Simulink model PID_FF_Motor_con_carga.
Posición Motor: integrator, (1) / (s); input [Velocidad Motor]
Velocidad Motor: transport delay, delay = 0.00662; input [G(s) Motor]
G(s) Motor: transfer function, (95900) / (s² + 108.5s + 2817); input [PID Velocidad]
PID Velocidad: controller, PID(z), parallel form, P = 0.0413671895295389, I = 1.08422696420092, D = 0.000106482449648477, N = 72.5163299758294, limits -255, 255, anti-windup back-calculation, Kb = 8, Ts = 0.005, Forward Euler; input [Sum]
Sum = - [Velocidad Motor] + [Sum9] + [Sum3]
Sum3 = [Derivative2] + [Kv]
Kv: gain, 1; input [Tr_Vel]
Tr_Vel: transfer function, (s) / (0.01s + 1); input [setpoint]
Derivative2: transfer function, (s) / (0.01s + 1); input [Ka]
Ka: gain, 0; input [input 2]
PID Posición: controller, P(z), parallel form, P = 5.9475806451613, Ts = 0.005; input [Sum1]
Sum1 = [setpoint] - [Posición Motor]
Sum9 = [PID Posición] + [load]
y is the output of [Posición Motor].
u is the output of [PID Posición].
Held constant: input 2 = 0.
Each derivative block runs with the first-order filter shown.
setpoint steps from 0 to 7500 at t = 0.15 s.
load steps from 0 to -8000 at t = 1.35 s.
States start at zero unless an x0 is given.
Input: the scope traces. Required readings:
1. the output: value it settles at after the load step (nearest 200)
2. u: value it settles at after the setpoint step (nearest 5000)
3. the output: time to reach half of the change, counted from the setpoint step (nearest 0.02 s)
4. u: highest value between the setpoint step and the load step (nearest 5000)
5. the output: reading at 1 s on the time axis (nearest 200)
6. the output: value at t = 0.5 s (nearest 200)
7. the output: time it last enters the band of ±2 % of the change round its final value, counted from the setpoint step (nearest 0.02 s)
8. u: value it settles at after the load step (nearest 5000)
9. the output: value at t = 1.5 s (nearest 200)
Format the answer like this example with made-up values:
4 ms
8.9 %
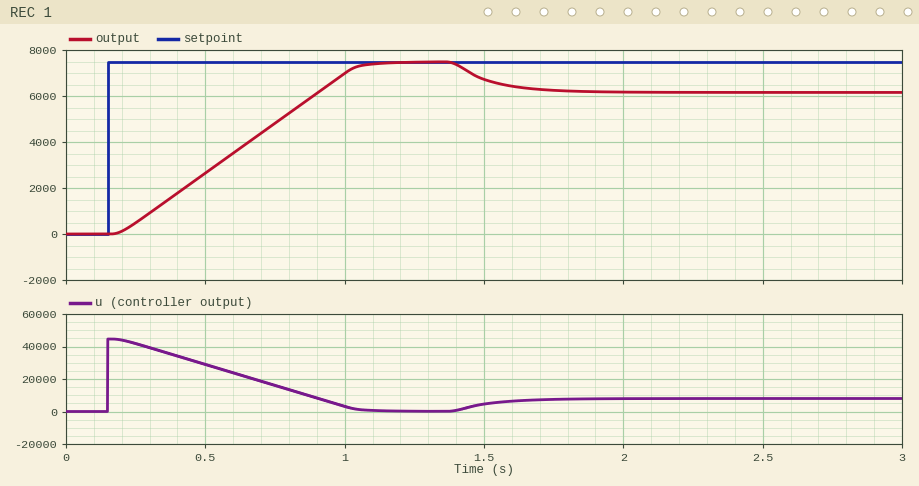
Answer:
6200
0
0.48 s
45000
7000
2600
0.92 s
10000
6800
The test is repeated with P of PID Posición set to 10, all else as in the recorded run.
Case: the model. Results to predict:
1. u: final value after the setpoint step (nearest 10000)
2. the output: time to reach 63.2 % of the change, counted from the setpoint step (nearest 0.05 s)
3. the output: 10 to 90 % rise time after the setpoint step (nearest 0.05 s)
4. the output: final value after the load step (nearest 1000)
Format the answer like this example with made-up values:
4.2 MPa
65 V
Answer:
0
0.60 s
0.70 s
7000
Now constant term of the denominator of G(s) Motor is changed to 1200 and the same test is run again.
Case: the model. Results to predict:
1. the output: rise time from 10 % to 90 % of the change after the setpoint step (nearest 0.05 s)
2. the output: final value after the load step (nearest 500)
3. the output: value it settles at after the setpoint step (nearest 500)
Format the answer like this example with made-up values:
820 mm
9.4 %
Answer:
0.30 s
6000
7500
